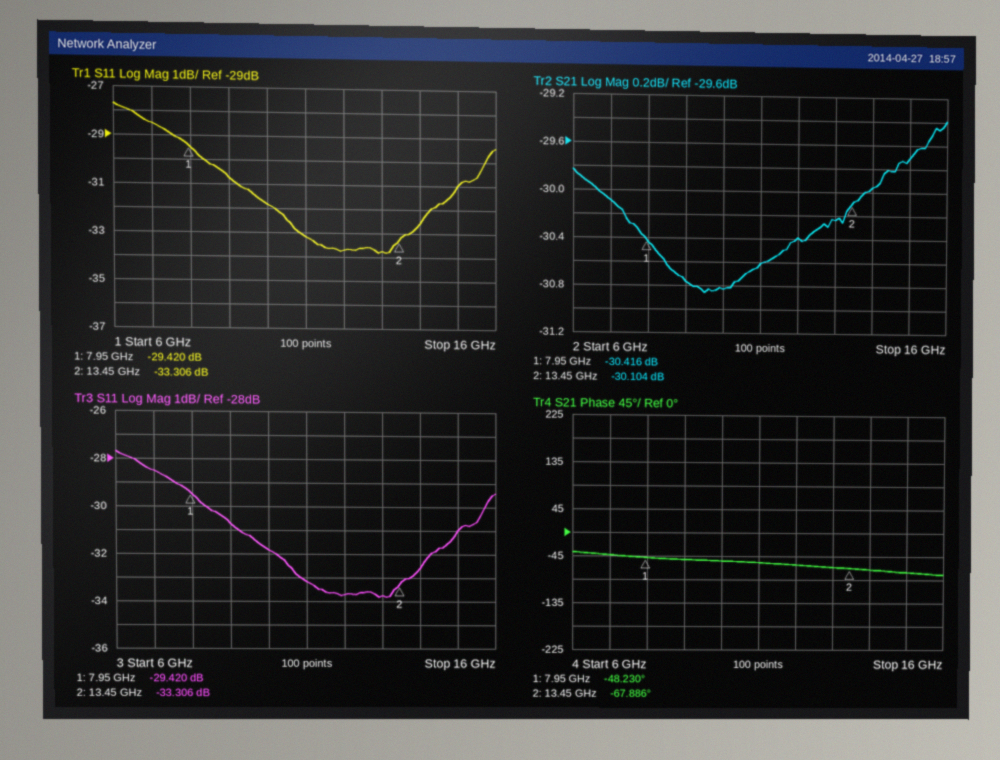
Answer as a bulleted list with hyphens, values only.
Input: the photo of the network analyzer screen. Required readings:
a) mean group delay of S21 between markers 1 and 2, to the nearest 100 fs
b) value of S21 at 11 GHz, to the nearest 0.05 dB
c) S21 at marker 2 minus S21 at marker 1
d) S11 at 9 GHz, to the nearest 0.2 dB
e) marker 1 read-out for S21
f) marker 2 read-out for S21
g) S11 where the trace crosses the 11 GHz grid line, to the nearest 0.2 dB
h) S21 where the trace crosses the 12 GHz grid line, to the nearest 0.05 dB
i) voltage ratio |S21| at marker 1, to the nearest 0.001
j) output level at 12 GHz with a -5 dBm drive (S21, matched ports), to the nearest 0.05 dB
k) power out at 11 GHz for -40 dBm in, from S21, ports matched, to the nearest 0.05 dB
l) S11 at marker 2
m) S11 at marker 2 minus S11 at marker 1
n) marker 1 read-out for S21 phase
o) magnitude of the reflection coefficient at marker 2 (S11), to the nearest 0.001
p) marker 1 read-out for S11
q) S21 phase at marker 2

- 9.9 ps
- -30.60 dB
- 0.312 dB
- -30.8 dB
- -30.416 dB
- -30.104 dB
- -33.2 dB
- -30.40 dB
- 0.030
- -35.40 dBm
- -70.60 dBm
- -33.306 dB
- -3.886 dB
- -48.230°
- 0.022
- -29.420 dB
- -67.886°
